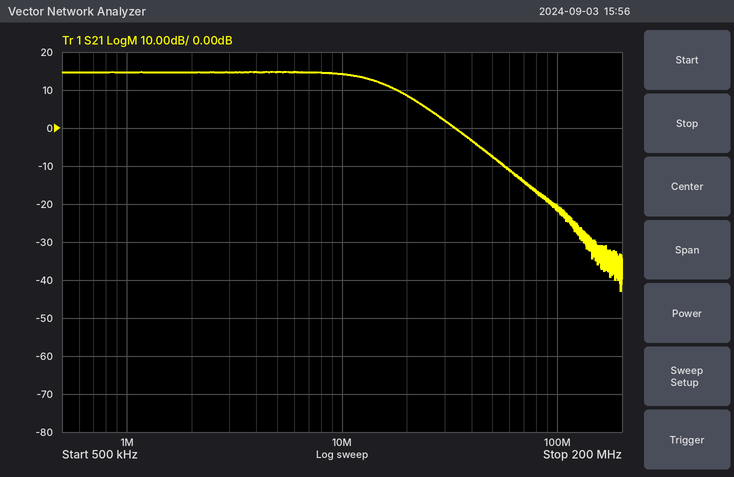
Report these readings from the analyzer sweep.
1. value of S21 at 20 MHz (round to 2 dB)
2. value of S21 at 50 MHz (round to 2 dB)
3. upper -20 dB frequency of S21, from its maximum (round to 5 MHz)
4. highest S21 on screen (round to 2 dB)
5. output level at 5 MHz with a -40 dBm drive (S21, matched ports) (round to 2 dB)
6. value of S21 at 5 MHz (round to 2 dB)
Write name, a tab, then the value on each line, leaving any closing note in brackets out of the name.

value of S21 at 20 MHz	8 dB
value of S21 at 50 MHz	-8 dB
upper -20 dB frequency of S21, from its maximum	45 MHz
highest S21 on screen	14 dB
output level at 5 MHz with a -40 dBm drive (S21, matched ports)	-26 dBm
value of S21 at 5 MHz	14 dB
